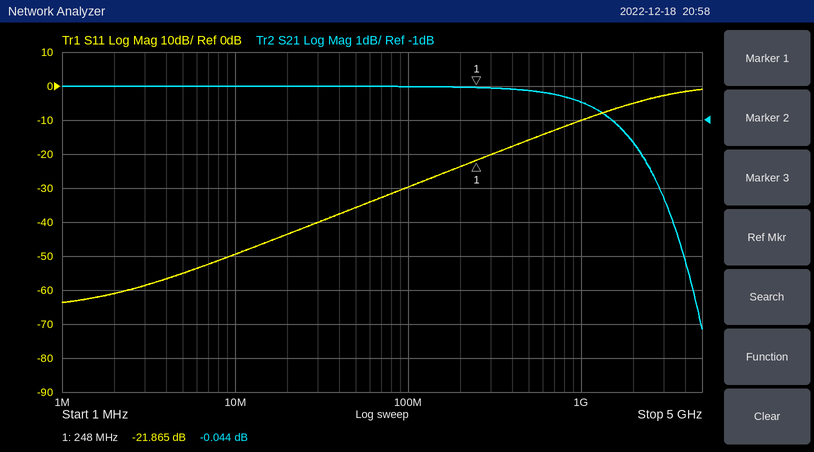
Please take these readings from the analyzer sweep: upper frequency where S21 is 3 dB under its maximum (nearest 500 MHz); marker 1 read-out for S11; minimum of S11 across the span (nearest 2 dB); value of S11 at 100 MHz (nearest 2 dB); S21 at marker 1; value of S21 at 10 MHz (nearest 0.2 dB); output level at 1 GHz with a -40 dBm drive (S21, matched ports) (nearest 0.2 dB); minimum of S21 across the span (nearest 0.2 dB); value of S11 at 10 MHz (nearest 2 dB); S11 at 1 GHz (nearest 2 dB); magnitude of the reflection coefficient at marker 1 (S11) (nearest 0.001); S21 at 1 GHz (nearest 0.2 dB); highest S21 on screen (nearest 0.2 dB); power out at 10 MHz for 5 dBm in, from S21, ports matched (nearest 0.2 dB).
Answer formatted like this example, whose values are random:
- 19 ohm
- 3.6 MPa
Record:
- 3.0 GHz
- -21.865 dB
- -64 dB
- -30 dB
- -0.044 dB
- 0.0 dB
- -40.4 dBm
- -7.2 dB
- -50 dB
- -10 dB
- 0.081
- -0.4 dB
- 0.0 dB
- 5.0 dBm
